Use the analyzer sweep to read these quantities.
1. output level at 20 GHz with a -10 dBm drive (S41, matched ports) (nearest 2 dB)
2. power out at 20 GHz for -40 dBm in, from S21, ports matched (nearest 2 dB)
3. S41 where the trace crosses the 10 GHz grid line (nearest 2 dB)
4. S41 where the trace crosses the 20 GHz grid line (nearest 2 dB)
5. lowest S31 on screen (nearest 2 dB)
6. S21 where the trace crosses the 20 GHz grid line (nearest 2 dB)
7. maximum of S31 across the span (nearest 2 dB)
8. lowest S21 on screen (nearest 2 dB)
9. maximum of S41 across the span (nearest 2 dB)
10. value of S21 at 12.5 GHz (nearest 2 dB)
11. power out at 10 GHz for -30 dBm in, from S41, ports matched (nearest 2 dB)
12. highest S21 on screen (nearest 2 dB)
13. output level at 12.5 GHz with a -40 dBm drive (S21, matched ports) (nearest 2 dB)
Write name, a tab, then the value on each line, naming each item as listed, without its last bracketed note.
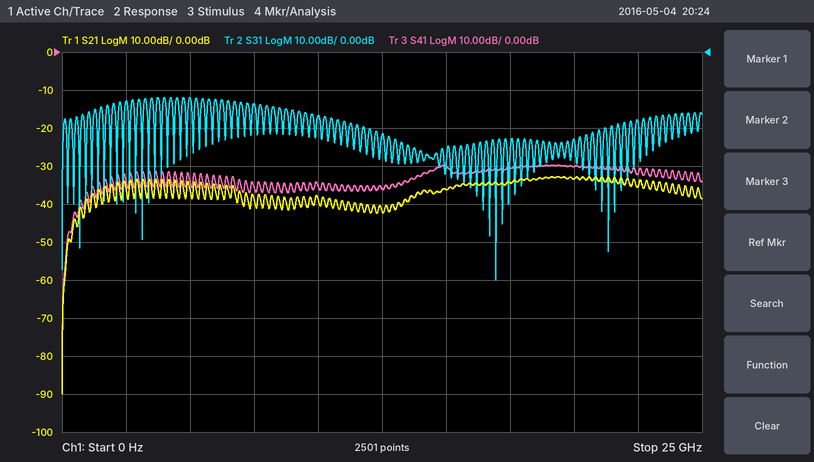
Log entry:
output level at 20 GHz with a -10 dBm drive (S41, matched ports)	-40 dBm
power out at 20 GHz for -40 dBm in, from S21, ports matched	-74 dBm
S41 where the trace crosses the 10 GHz grid line	-36 dB
S41 where the trace crosses the 20 GHz grid line	-30 dB
lowest S31 on screen	-60 dB
S21 where the trace crosses the 20 GHz grid line	-34 dB
maximum of S31 across the span	-12 dB
lowest S21 on screen	-90 dB
maximum of S41 across the span	-30 dB
value of S21 at 12.5 GHz	-42 dB
power out at 10 GHz for -30 dBm in, from S41, ports matched	-66 dBm
highest S21 on screen	-32 dB
output level at 12.5 GHz with a -40 dBm drive (S21, matched ports)	-82 dBm
